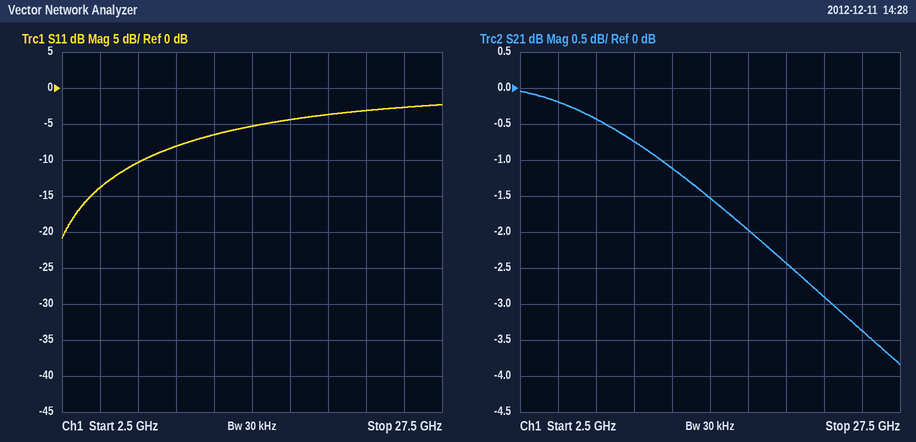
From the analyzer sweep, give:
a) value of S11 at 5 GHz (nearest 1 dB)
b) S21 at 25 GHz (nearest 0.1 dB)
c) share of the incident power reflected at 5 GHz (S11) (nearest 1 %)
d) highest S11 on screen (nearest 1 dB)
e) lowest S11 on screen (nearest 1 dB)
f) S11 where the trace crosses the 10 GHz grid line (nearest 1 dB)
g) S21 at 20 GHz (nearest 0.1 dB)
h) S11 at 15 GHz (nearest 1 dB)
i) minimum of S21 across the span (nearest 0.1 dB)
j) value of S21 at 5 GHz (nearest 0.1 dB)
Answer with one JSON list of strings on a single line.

["-14 dB", "-3.4 dB", "4 %", "-2 dB", "-21 dB", "-8 dB", "-2.4 dB", "-5 dB", "-3.8 dB", "-0.2 dB"]
